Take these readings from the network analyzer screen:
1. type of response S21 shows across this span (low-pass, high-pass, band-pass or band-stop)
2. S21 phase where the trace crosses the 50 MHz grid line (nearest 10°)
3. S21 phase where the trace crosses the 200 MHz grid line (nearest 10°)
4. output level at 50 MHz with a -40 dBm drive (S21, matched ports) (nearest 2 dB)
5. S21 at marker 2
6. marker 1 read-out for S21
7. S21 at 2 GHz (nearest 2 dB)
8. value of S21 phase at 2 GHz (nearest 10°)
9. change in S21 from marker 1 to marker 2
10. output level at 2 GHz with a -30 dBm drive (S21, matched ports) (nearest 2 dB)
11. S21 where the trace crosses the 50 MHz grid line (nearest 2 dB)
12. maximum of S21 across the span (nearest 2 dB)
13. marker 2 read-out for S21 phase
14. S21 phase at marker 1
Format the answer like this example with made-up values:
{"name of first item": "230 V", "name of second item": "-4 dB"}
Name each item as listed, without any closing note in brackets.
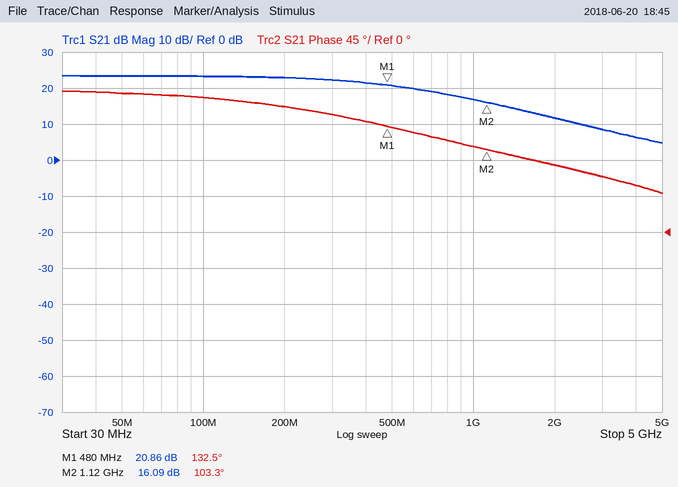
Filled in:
{"type of response S21 shows across this span": "low-pass", "S21 phase where the trace crosses the 50 MHz grid line": "170°", "S21 phase where the trace crosses the 200 MHz grid line": "160°", "output level at 50 MHz with a -40 dBm drive (S21, matched ports)": "-16 dBm", "S21 at marker 2": "16.09 dB", "marker 1 read-out for S21": "20.86 dB", "S21 at 2 GHz": "12 dB", "value of S21 phase at 2 GHz": "80°", "change in S21 from marker 1 to marker 2": "-4.77 dB", "output level at 2 GHz with a -30 dBm drive (S21, matched ports)": "-18 dBm", "S21 where the trace crosses the 50 MHz grid line": "24 dB", "maximum of S21 across the span": "24 dB", "marker 2 read-out for S21 phase": "103.3°", "S21 phase at marker 1": "132.5°"}
